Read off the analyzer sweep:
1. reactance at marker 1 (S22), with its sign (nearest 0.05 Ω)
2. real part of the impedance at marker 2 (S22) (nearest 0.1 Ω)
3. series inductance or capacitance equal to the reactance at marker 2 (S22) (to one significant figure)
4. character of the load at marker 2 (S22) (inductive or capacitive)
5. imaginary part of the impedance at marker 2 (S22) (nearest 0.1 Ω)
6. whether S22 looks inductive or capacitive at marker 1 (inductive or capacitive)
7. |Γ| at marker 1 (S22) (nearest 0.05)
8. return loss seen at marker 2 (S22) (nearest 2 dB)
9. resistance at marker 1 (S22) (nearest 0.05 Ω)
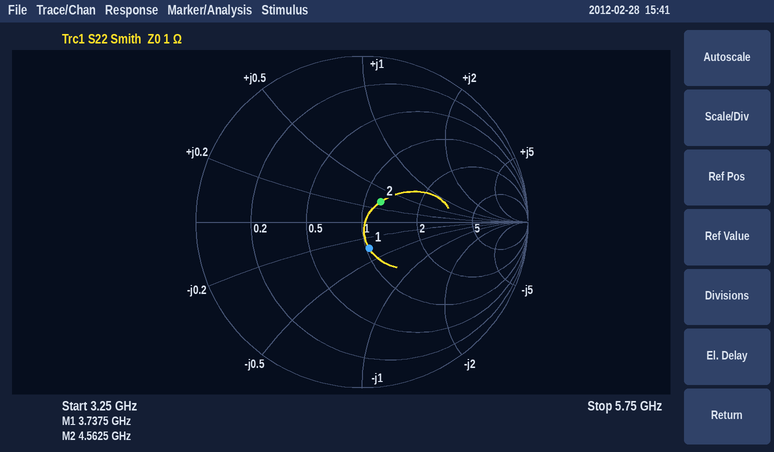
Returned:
-0.35 Ω
1.2 Ω
10 pH
inductive
+0.3 Ω
capacitive
0.15
16 dB
1.05 Ω
